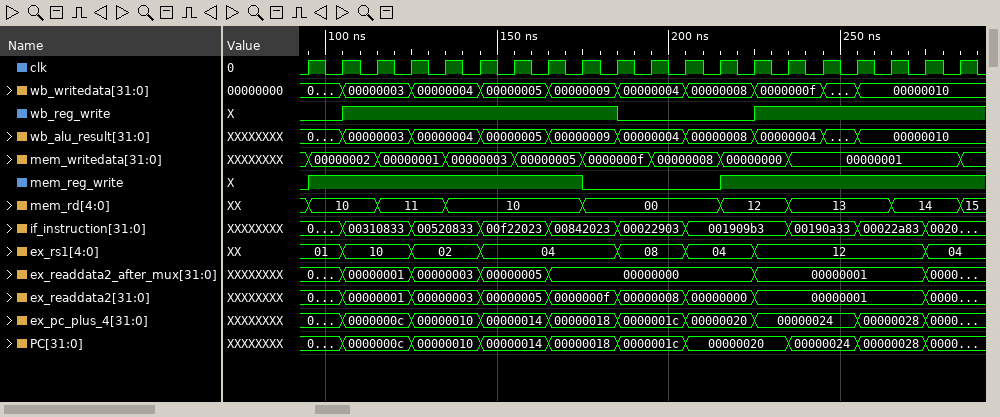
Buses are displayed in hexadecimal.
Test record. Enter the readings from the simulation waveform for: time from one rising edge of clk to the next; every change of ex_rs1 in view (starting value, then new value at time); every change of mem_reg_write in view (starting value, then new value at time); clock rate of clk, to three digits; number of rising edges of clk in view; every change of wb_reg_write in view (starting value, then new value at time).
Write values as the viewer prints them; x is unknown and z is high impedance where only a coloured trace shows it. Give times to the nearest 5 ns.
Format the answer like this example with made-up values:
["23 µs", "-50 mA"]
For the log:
["10 ns", "01, 10 at 105 ns, 02 at 125 ns, 04 at 145 ns, 08 at 185 ns, 04 at 205 ns, 12 at 225 ns, 04 at 275 ns", "0, 1 at 95 ns, 0 at 175 ns, 1 at 215 ns", "100 MHz", "20", "0, 1 at 105 ns, 0 at 185 ns, 1 at 225 ns"]
